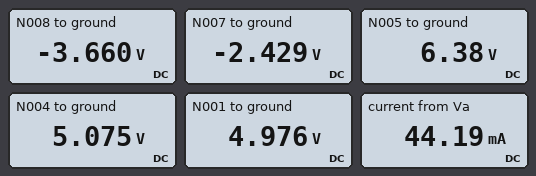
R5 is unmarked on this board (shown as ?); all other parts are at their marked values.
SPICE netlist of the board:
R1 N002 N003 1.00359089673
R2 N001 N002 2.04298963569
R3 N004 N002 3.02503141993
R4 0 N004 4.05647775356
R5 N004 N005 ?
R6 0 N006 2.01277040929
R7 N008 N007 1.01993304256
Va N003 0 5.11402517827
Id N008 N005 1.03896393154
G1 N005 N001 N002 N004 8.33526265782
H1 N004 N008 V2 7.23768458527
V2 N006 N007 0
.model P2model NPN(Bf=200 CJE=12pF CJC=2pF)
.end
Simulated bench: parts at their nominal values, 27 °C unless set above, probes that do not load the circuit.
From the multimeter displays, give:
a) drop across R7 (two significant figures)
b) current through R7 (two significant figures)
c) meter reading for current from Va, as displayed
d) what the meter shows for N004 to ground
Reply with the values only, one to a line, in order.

1.2 V
1.2 A
44.19 mA
5.075 V
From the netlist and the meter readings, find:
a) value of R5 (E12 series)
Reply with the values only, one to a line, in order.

1.2 Ω
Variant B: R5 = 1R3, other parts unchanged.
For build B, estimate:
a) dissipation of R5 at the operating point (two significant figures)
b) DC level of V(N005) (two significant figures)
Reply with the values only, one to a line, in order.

1.5 W
6.5 V
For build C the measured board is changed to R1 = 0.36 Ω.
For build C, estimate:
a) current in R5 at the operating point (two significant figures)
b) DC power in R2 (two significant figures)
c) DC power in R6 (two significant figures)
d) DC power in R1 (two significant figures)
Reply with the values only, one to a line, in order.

1.1 A
4.4 mW
3.0 W
710 µW
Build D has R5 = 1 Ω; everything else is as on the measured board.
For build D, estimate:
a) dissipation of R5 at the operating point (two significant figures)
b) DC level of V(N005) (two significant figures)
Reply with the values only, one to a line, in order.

1.2 W
6.2 V
